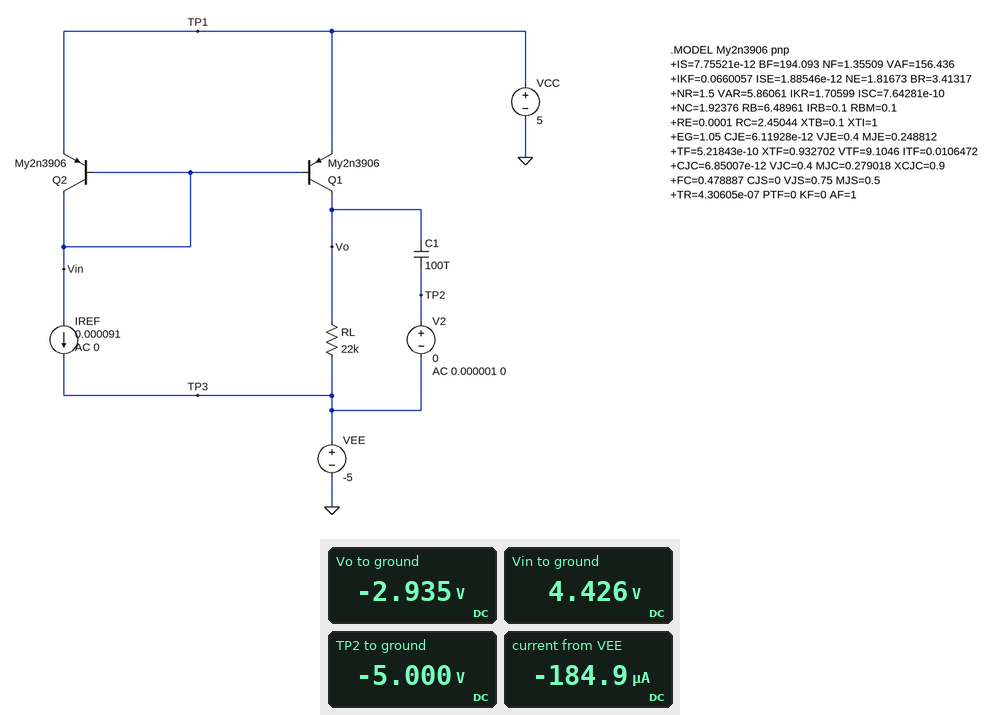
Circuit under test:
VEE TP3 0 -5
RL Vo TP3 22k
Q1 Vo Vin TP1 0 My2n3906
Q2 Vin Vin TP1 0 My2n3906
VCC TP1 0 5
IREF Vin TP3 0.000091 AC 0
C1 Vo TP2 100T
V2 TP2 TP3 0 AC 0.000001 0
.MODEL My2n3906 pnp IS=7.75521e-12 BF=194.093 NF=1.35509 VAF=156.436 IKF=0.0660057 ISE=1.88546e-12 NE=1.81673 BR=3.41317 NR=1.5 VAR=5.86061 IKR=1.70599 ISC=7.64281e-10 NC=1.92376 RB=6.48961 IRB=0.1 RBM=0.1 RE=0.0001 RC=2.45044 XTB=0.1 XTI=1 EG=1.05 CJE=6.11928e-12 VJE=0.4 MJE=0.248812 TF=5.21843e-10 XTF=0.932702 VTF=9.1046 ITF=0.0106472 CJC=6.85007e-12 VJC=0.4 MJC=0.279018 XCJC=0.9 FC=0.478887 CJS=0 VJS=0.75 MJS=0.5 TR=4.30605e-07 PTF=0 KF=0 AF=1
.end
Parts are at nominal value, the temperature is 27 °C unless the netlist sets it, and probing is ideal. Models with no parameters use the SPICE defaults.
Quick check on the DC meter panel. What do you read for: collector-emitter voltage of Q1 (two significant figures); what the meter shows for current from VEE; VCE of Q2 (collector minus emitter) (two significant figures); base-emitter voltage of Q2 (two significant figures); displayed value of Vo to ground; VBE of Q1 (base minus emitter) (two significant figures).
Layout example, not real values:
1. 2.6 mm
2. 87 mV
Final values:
1. -7.9 V
2. -184.9 µA
3. -570 mV
4. -570 mV
5. -2.935 V
6. -570 mV
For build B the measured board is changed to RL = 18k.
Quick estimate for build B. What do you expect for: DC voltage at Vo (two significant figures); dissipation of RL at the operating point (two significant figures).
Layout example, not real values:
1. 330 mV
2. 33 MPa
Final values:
1. -3.3 V
2. 160 µW
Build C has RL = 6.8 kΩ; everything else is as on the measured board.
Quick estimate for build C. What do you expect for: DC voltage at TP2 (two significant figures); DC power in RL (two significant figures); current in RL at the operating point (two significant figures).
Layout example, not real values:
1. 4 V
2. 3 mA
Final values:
1. -5.0 V
2. 61 µW
3. 95 µA
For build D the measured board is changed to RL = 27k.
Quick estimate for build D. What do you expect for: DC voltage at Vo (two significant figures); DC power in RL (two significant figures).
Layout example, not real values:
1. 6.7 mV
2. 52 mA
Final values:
1. -2.5 V
2. 240 µW
